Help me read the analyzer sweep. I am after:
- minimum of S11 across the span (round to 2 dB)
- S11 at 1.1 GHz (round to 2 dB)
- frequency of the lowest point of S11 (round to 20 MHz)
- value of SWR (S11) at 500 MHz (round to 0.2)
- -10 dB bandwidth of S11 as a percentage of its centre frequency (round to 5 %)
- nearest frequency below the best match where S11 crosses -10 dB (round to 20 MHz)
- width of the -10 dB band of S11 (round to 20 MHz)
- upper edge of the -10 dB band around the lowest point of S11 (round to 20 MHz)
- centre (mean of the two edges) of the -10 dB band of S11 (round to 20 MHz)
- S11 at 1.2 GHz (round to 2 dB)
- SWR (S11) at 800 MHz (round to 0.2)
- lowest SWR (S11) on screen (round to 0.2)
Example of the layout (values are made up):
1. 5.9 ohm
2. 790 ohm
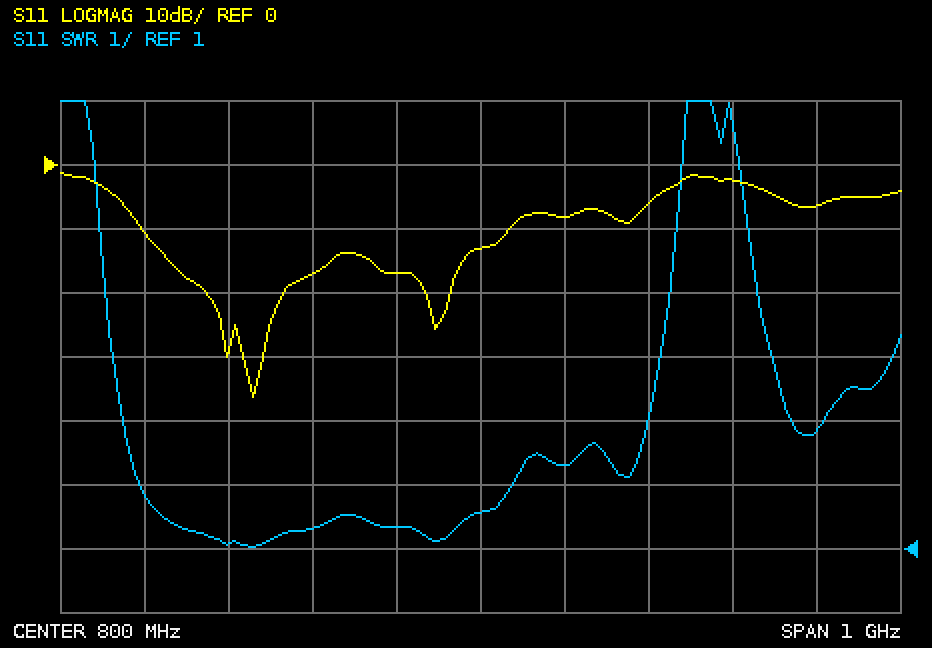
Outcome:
1. -36 dB
2. -2 dB
3. 520 MHz
4. 1.0
5. 70 %
6. 400 MHz
7. 440 MHz
8. 840 MHz
9. 620 MHz
10. -6 dB
11. 1.6
12. 1.0
